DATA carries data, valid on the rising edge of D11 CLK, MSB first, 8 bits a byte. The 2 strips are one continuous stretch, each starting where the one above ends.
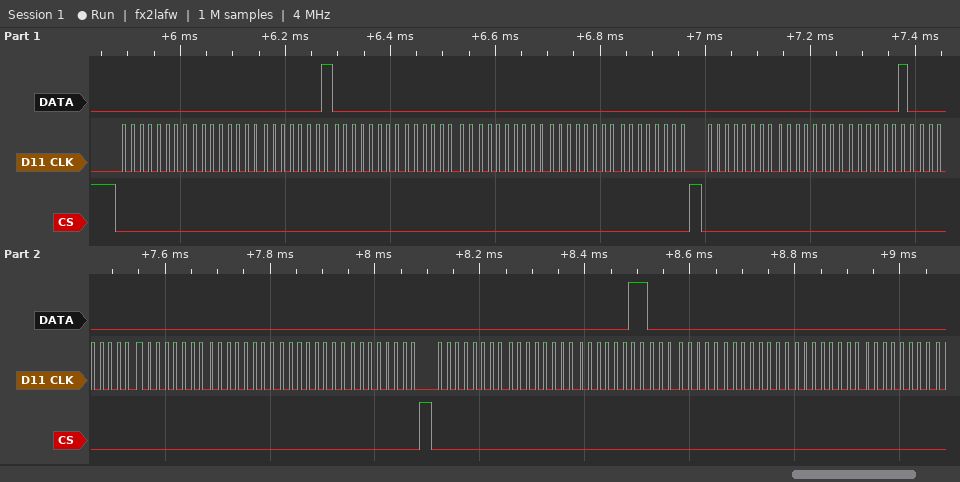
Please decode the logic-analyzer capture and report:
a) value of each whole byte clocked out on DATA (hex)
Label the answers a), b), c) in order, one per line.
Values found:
a) 0x00 0x00 0x01 0x00 0x00 0x00 0x00 0x00 0x00 0x00 0x02 0x00 0x00 0x00 0x00 0x00 0x00 0x00 0x03 0x00 0x00 0x00 0x00
